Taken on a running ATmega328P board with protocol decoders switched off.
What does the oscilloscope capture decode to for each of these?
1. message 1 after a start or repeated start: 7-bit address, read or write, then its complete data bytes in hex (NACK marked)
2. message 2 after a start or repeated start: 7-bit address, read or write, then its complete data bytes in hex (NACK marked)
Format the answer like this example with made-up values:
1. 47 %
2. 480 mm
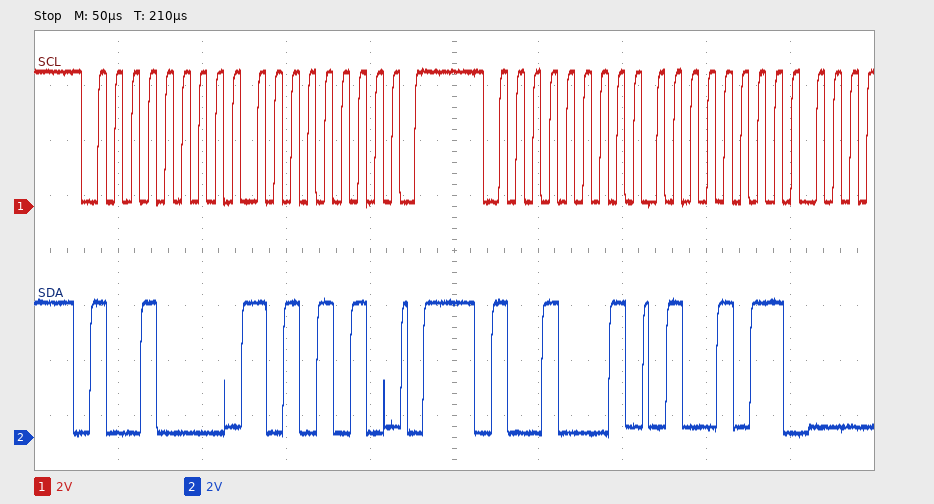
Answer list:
1. 0x48 write: AA
2. 0x48 read: 4B
